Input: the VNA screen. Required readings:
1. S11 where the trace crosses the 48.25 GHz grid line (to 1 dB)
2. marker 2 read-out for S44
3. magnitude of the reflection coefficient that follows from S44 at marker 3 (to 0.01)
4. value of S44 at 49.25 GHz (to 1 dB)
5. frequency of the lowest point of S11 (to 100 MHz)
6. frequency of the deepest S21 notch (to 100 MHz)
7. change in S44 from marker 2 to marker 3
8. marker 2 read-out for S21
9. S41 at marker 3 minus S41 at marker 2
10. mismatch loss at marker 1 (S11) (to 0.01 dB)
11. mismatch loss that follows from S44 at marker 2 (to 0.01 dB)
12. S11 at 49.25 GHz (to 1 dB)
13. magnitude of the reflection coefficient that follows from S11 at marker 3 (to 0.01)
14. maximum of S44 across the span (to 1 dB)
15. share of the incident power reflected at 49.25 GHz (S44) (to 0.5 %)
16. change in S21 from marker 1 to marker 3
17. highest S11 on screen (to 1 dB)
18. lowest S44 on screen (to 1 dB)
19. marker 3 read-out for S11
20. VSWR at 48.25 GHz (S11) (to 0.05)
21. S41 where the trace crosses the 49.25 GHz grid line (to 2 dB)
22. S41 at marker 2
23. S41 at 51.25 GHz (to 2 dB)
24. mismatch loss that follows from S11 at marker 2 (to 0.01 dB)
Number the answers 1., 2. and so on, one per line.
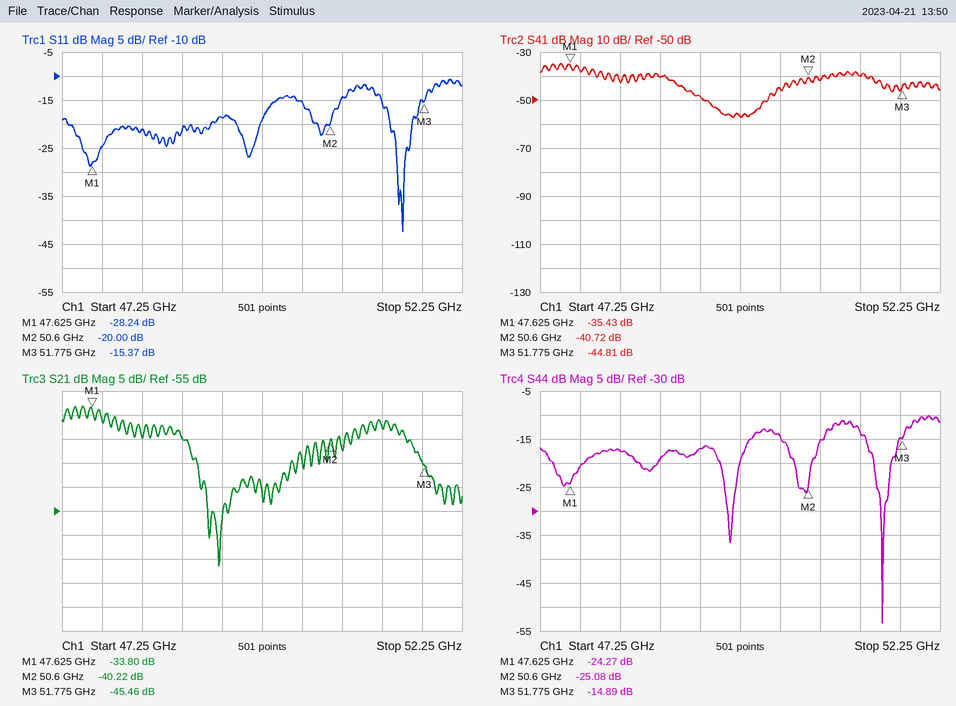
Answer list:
1. -21 dB
2. -25.08 dB
3. 0.18
4. -17 dB
5. 51.5 GHz
6. 49.2 GHz
7. 10.19 dB
8. -40.22 dB
9. -4.09 dB
10. 0.01 dB
11. 0.01 dB
12. -19 dB
13. 0.17
14. -10 dB
15. 2.0 %
16. -11.66 dB
17. -11 dB
18. -53 dB
19. -15.37 dB
20. 1.20
21. -48 dB
22. -40.72 dB
23. -40 dB
24. 0.04 dB
